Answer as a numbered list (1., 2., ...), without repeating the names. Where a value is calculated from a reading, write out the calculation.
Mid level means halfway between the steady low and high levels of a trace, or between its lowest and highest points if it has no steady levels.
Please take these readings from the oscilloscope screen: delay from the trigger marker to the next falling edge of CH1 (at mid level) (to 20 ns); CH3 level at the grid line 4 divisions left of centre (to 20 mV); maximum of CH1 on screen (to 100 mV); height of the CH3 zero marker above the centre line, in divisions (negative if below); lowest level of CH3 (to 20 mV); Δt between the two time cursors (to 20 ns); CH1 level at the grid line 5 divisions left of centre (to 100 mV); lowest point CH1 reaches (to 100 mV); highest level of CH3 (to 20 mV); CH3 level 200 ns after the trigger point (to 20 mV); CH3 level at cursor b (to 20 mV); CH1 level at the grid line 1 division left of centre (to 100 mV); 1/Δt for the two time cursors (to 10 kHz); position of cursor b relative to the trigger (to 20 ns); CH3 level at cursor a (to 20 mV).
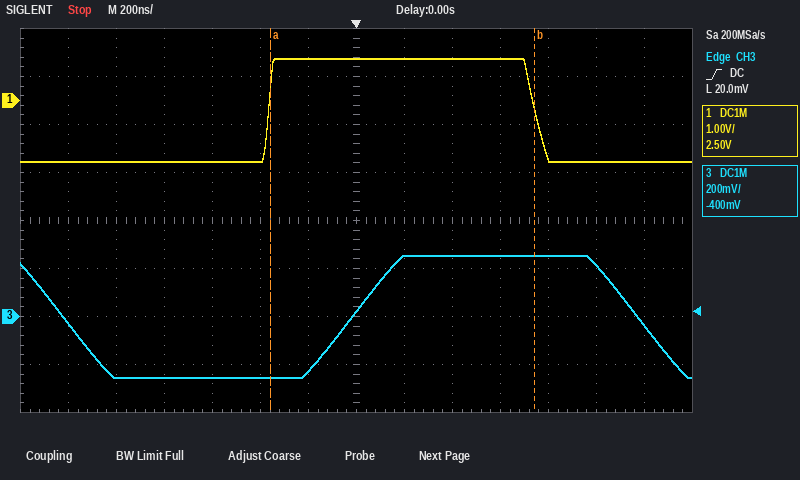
1. 740 ns
2. -260 mV
3. 900 mV
4. -2.0 div
5. -260 mV
6. 1.10 µs
7. -1.3 V
8. -1.3 V
9. 260 mV
10. 260 mV
11. 260 mV
12. 900 mV
13. 1 / 1.10 µs ≈ 910 kHz
14. +740 ns
15. -260 mV
